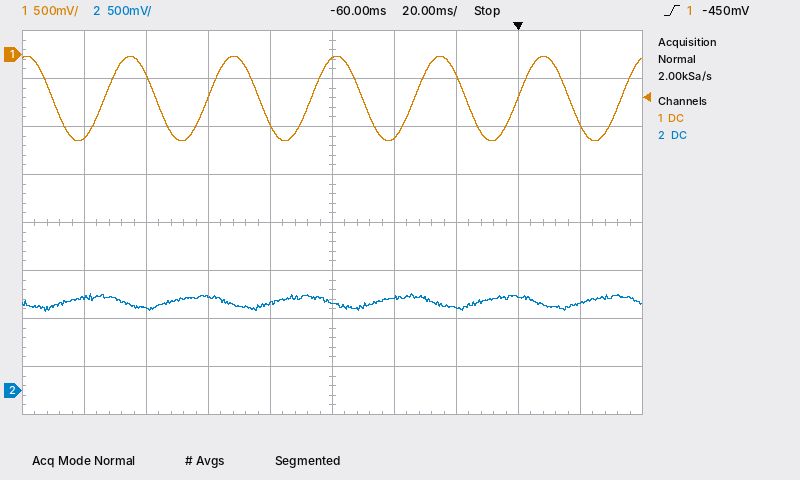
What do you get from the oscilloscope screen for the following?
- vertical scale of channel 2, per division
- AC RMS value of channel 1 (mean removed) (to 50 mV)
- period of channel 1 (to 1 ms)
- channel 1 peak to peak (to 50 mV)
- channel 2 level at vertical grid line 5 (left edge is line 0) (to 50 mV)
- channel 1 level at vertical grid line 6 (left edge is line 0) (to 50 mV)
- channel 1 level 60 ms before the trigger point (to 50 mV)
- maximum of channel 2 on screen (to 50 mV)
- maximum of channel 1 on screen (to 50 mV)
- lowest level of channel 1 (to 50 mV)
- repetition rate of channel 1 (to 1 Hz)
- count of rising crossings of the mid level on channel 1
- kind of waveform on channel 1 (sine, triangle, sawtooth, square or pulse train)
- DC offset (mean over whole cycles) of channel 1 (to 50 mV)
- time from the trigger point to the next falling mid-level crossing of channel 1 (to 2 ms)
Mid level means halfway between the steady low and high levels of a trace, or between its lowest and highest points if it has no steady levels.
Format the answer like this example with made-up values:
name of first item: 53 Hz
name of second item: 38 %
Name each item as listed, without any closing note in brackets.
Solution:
vertical scale of channel 2, per division: 500 mV
AC RMS value of channel 1 (mean removed): 300 mV
period of channel 1: 33 ms
channel 1 peak to peak: 900 mV
channel 2 level at vertical grid line 5 (left edge is line 0): 900 mV
channel 1 level at vertical grid line 6 (left edge is line 0): -850 mV
channel 1 level 60 ms before the trigger point: -50 mV
maximum of channel 2 on screen: 1.00 V
maximum of channel 1 on screen: 0 mV
lowest level of channel 1: -900 mV
repetition rate of channel 1: 30 Hz
count of rising crossings of the mid level on channel 1: 6
kind of waveform on channel 1: sine
DC offset (mean over whole cycles) of channel 1: -450 mV
time from the trigger point to the next falling mid-level crossing of channel 1: 16 ms
